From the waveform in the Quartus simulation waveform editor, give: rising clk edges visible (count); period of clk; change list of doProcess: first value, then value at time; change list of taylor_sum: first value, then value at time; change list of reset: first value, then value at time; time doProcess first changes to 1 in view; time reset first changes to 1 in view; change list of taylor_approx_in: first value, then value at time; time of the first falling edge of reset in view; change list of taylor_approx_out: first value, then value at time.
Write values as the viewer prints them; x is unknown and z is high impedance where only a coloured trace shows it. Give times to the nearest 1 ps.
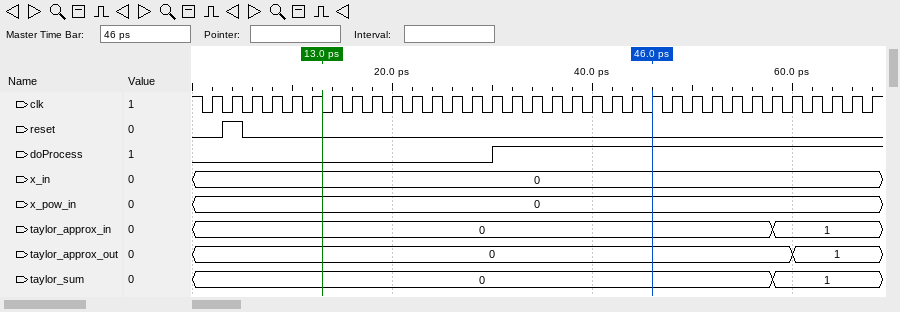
34
2 ps
0, 1 at 30 ps
0, 1 at 58 ps
0, 1 at 3 ps, 0 at 5 ps
30 ps
3 ps
0, 1 at 58 ps
5 ps
0, 1 at 60 ps
